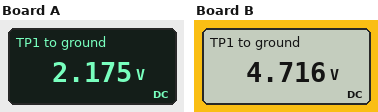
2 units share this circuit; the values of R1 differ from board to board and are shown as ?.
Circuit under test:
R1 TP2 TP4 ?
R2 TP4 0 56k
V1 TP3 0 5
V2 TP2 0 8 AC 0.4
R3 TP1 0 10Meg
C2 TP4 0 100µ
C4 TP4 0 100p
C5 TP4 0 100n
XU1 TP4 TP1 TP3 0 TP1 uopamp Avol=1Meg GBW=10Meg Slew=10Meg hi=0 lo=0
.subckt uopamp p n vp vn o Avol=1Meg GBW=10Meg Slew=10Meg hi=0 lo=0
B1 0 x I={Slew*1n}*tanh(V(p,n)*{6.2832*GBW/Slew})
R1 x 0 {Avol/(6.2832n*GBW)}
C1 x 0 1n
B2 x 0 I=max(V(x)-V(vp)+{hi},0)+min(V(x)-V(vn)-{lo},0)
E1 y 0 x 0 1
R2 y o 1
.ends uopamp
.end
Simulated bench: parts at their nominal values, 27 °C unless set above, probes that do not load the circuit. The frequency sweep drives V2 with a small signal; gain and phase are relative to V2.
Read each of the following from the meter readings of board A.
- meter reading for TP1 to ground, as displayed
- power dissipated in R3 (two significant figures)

2.175 V
470 nW
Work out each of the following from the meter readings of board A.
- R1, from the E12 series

150 kΩ
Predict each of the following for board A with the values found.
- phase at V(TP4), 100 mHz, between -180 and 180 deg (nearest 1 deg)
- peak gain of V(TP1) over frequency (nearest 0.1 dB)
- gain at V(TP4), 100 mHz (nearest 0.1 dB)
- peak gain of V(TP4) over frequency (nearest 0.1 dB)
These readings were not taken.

-69 deg
-11.3 dB
-20.1 dB
-11.3 dB
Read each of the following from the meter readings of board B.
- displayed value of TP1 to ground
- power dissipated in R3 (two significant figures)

4.716 V
2.2 µW
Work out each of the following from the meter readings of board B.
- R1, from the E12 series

39 kΩ
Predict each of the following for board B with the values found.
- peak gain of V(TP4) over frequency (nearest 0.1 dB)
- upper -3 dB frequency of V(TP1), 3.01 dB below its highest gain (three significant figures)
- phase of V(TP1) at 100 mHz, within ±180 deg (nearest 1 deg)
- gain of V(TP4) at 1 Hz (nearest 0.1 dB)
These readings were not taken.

-4.6 dB
69.2 mHz
-55 deg
-27.8 dB
